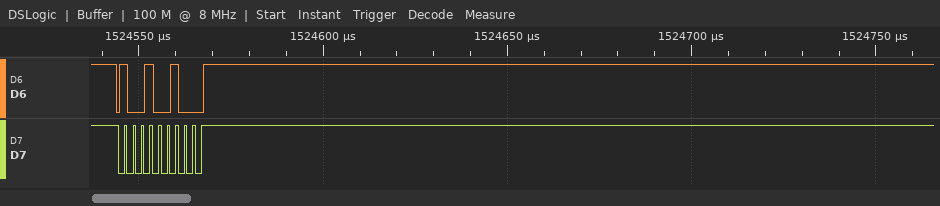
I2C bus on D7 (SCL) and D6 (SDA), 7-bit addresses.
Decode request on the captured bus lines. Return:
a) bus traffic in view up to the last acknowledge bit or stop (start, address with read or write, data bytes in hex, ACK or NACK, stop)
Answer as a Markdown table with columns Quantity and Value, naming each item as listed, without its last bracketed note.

| Quantity | Value |
|---|---|
| bus traffic in view up to the last acknowledge bit or stop | start, address 49 write ACK, stop |
